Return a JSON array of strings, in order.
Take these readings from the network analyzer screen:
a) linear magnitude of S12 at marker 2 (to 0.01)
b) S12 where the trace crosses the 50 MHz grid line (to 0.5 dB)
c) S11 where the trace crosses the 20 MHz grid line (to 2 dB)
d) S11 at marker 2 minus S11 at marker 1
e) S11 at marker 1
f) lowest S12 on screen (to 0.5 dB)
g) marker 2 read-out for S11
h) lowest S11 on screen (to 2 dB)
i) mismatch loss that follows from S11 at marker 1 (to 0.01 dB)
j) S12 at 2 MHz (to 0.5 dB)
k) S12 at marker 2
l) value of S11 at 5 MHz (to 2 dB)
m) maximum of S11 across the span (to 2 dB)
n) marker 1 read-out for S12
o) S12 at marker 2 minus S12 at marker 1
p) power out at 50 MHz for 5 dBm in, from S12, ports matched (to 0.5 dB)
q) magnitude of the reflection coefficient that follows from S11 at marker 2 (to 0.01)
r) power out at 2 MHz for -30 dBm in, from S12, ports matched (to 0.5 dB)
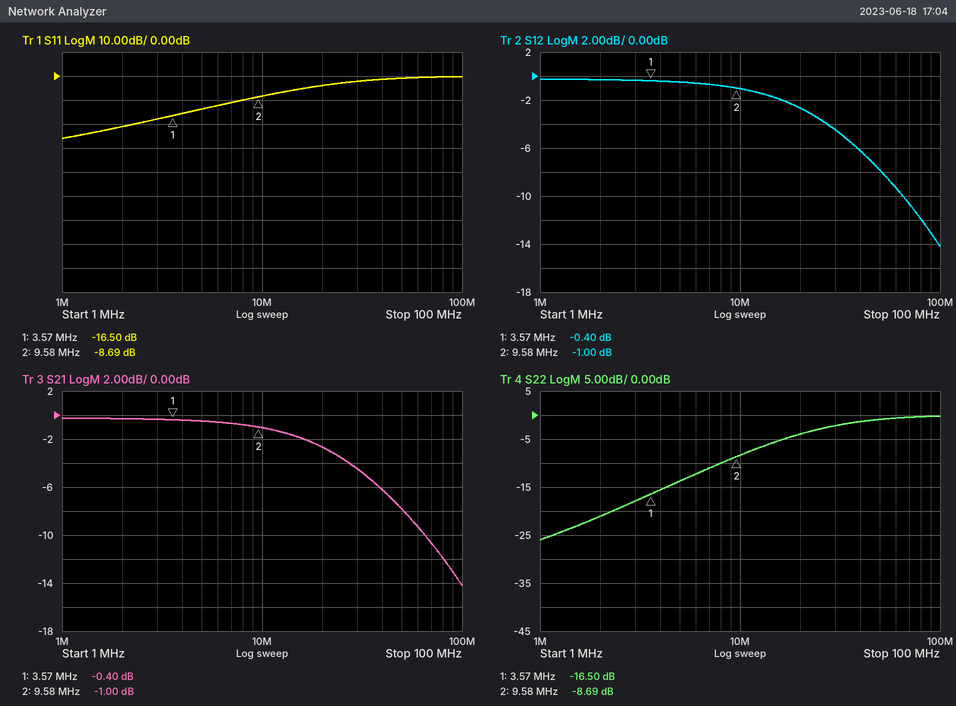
["0.89", "-8.0 dB", "-4 dB", "7.81 dB", "-16.50 dB", "-14.0 dB", "-8.69 dB", "-26 dB", "0.10 dB", "-0.5 dB", "-1.00 dB", "-14 dB", "0 dB", "-0.40 dB", "-0.60 dB", "-3.0 dBm", "0.37", "-30.5 dBm"]
